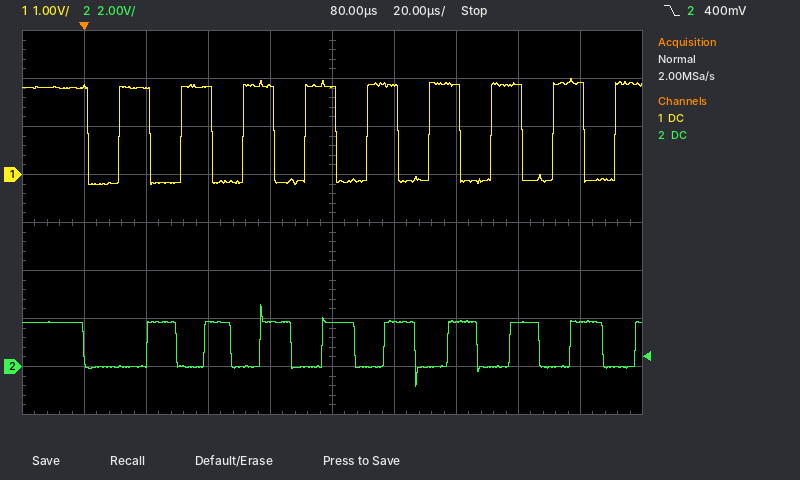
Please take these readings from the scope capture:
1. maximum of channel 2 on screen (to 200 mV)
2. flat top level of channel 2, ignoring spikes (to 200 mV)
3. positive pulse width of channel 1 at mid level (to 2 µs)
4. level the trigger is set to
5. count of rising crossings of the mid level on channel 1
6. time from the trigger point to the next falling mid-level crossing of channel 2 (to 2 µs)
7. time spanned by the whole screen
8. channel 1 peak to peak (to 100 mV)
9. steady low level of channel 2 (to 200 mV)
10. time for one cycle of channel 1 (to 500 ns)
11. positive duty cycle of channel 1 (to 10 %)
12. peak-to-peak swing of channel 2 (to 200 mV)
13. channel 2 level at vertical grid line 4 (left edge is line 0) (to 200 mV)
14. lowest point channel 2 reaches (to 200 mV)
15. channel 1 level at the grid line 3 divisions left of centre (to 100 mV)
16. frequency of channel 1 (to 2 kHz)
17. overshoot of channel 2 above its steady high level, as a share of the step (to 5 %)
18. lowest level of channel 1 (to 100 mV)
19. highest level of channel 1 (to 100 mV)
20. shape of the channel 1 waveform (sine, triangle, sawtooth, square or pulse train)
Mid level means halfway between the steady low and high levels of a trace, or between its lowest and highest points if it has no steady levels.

2.6 V
1.8 V
10 µs
400 mV
9
30 µs
200 µs
2.2 V
0.0 V
20.0 µs
50 %
3.4 V
1.8 V
-800 mV
1.8 V
50 kHz
40 %
-200 mV
2.0 V
square
